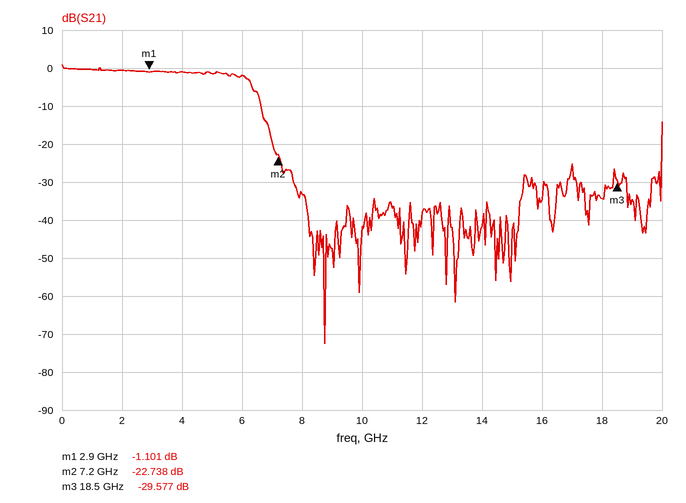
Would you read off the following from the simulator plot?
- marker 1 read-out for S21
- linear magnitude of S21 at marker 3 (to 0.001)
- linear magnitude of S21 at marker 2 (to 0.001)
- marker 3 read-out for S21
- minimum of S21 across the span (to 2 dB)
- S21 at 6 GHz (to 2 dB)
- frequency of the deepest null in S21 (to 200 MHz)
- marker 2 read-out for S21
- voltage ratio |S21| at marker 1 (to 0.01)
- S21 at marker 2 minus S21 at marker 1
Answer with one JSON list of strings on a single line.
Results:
["-1.101 dB", "0.033", "0.073", "-29.577 dB", "-72 dB", "-2 dB", "8.8 GHz", "-22.738 dB", "0.88", "-21.637 dB"]
